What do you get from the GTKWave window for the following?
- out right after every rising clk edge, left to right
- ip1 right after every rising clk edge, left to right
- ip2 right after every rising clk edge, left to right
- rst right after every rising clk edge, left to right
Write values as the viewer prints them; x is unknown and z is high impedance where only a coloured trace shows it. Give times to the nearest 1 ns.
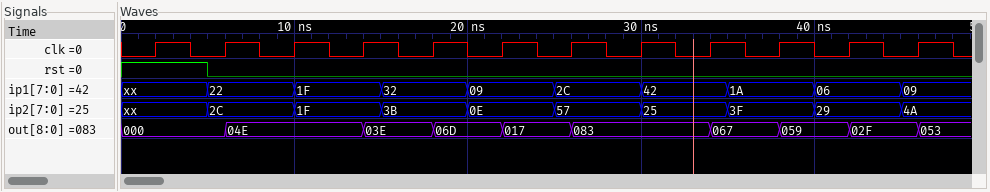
000, 04E, 04E, 03E, 06D, 017, 083, 083, 067, 059, 02F, 053
xx, 22, 1F, 1F, 32, 09, 2C, 42, 42, 1A, 06, 09
xx, 2C, 1F, 1F, 3B, 0E, 57, 25, 25, 3F, 29, 4A
1 0 0 0 0 0 0 0 0 0 0 0
